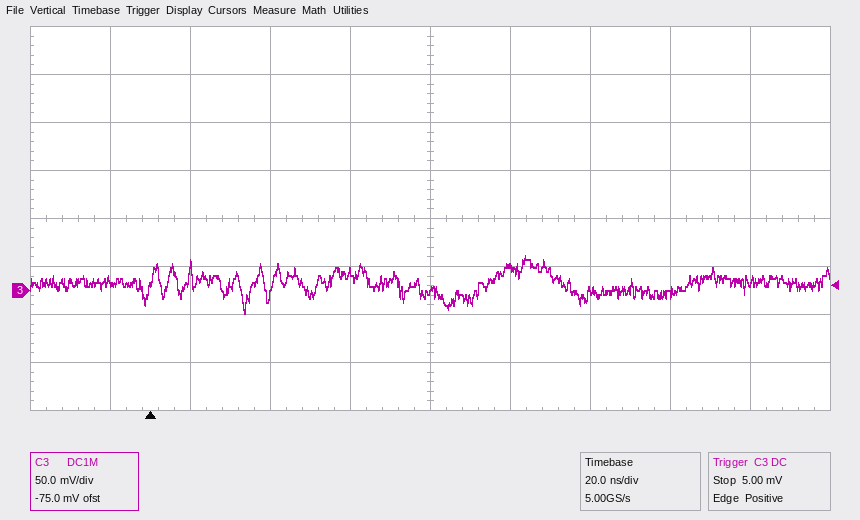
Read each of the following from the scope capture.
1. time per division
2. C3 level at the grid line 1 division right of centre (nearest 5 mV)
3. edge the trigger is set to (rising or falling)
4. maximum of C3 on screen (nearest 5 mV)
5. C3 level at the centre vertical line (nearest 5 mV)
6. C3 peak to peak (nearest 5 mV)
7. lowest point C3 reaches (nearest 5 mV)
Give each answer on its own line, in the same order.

20 ns
25 mV
rising
35 mV
0 mV
60 mV
-25 mV
